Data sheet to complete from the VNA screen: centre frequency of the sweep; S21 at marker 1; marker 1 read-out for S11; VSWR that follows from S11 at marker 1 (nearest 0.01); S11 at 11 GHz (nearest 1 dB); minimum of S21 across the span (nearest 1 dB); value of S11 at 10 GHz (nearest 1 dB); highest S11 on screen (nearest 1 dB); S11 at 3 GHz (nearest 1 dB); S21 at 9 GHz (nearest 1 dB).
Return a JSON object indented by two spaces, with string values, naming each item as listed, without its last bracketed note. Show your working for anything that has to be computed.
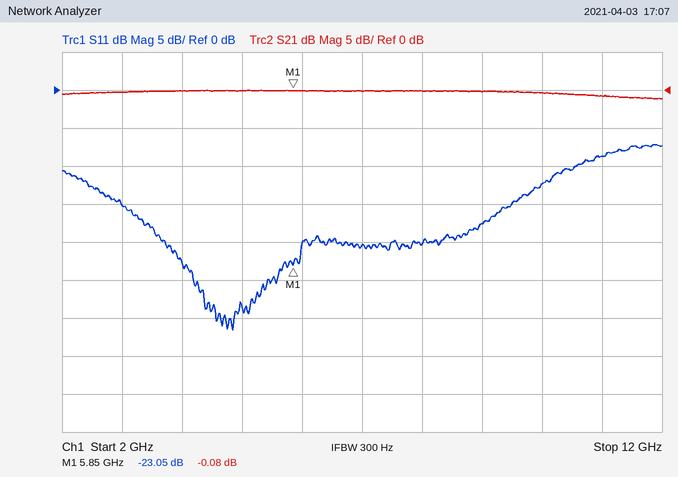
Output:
{
  "centre frequency of the sweep": "7 GHz",
  "S21 at marker 1": "-0.08 dB",
  "marker 1 read-out for S11": "-23.05 dB",
  "VSWR that follows from S11 at marker 1": "(1 + 0.0704)/(1 − 0.0704) ≈ 1.15",
  "S11 at 11 GHz": "-9 dB",
  "minimum of S21 across the span": "-1 dB",
  "value of S11 at 10 GHz": "-12 dB",
  "highest S11 on screen": "-7 dB",
  "S11 at 3 GHz": "-15 dB",
  "S21 at 9 GHz": "0 dB"
}
